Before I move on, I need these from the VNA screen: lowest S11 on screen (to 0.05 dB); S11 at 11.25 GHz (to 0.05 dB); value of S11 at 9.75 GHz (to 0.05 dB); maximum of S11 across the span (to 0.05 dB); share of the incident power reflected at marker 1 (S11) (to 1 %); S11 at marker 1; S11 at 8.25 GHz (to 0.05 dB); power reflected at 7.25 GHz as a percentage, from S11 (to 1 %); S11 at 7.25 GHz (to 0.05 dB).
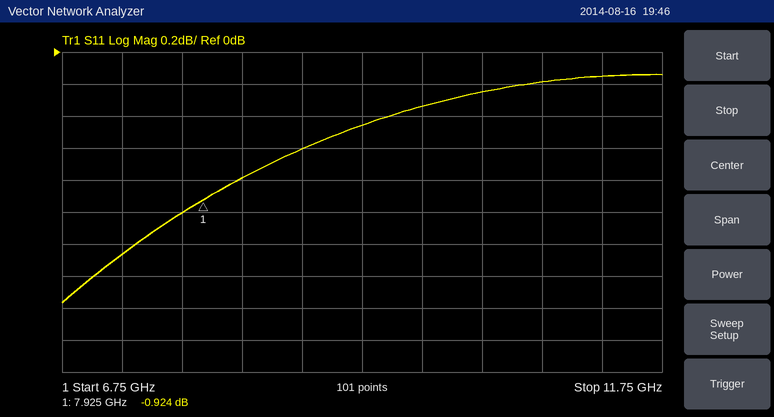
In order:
-1.55 dB
-0.15 dB
-0.35 dB
-0.15 dB
81 %
-0.924 dB
-0.80 dB
75 %
-1.25 dB
